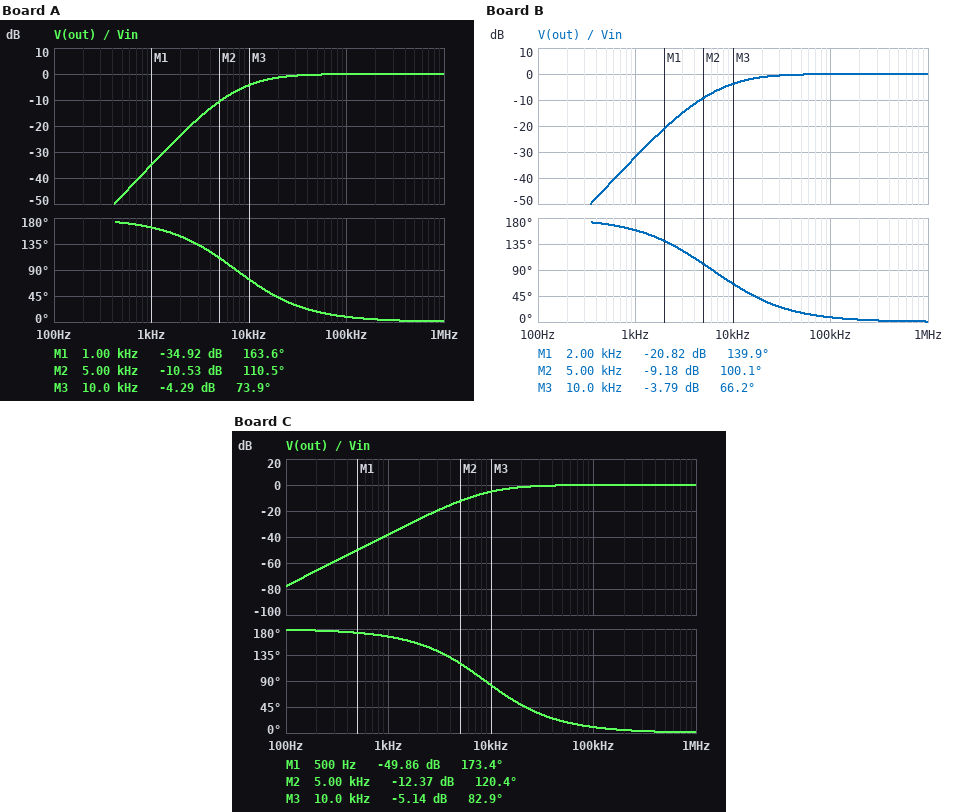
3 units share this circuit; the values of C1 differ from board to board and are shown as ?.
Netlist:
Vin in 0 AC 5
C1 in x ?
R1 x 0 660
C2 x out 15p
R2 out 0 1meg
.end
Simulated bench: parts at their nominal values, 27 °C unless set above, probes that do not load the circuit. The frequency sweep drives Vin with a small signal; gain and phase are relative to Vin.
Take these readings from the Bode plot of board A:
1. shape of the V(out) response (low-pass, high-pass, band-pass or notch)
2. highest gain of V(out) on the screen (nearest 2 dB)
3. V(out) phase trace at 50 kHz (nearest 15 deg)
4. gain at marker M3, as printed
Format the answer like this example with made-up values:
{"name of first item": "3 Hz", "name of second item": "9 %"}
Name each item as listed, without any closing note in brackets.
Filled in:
{"shape of the V(out) response": "high-pass", "highest gain of V(out) on the screen": "0 dB", "V(out) phase trace at 50 kHz": "15 deg", "gain at marker M3, as printed": "-4.29 dB"}
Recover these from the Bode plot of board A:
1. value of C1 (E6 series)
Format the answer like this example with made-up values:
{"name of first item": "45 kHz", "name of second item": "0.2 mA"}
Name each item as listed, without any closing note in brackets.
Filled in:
{"value of C1": "47 nF"}
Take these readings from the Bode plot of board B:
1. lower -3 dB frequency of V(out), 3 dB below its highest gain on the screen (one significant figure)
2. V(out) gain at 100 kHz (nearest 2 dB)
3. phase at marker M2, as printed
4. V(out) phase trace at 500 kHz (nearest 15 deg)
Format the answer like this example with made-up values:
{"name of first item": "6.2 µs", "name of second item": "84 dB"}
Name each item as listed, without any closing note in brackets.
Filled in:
{"lower -3 dB frequency of V(out), 3 dB below its highest gain on the screen": "10 kHz", "V(out) gain at 100 kHz": "0 dB", "phase at marker M2, as printed": "100.1 deg", "V(out) phase trace at 500 kHz": "0 deg"}
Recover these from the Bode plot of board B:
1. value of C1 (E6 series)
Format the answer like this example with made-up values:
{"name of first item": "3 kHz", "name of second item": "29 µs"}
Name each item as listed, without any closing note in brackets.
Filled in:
{"value of C1": "68 nF"}
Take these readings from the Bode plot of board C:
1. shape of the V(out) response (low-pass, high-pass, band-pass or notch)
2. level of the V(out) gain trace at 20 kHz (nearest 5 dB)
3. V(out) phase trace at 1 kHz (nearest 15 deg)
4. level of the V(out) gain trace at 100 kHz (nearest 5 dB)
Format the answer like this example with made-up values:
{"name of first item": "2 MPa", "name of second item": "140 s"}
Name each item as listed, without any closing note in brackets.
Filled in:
{"shape of the V(out) response": "high-pass", "level of the V(out) gain trace at 20 kHz": "0 dB", "V(out) phase trace at 1 kHz": "165 deg", "level of the V(out) gain trace at 100 kHz": "0 dB"}
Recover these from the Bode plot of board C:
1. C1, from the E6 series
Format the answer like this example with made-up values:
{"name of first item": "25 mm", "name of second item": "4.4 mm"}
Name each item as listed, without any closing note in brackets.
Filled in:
{"C1, from the E6 series": "33 nF"}
